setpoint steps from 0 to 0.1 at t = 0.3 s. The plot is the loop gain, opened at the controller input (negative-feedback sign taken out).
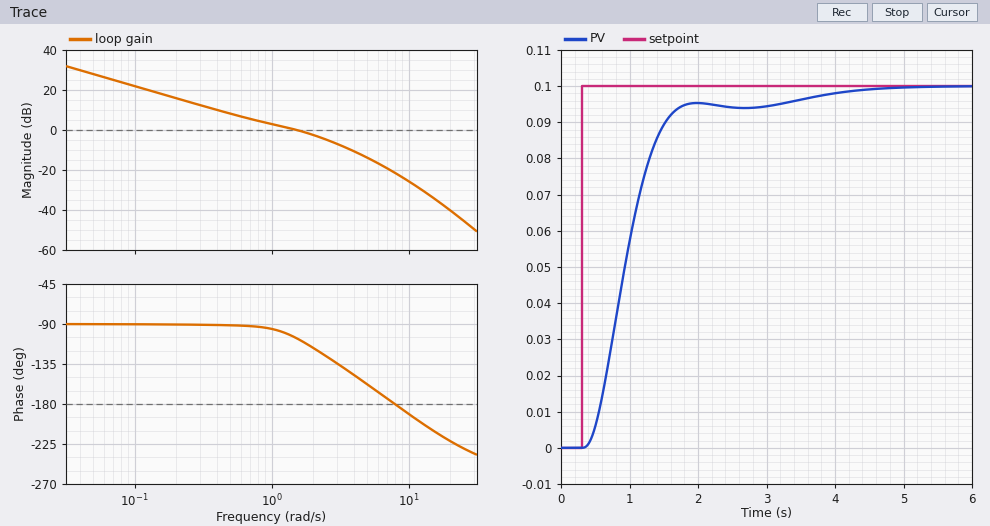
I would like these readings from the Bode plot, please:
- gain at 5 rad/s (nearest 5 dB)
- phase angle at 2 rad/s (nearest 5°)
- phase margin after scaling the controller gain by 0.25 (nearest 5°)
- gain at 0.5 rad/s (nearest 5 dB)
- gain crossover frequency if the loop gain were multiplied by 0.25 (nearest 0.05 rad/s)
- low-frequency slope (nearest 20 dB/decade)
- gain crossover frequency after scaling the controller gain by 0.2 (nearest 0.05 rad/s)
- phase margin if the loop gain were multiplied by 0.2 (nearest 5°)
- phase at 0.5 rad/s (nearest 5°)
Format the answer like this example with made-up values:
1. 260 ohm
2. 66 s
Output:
1. -15 dB
2. -115°
3. 90°
4. 10 dB
5. 0.30 rad/s
6. -20 dB/decade
7. 0.25 rad/s
8. 90°
9. -90°
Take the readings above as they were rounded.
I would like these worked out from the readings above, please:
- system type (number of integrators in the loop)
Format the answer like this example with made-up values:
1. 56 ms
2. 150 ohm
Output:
1. 1
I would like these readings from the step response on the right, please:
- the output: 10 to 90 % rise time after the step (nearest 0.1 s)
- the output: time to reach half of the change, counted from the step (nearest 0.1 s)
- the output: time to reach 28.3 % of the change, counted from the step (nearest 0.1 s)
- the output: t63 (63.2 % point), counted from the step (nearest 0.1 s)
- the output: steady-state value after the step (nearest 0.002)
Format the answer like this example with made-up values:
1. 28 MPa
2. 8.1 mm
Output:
1. 1.0 s
2. 0.6 s
3. 0.4 s
4. 0.8 s
5. 0.100
